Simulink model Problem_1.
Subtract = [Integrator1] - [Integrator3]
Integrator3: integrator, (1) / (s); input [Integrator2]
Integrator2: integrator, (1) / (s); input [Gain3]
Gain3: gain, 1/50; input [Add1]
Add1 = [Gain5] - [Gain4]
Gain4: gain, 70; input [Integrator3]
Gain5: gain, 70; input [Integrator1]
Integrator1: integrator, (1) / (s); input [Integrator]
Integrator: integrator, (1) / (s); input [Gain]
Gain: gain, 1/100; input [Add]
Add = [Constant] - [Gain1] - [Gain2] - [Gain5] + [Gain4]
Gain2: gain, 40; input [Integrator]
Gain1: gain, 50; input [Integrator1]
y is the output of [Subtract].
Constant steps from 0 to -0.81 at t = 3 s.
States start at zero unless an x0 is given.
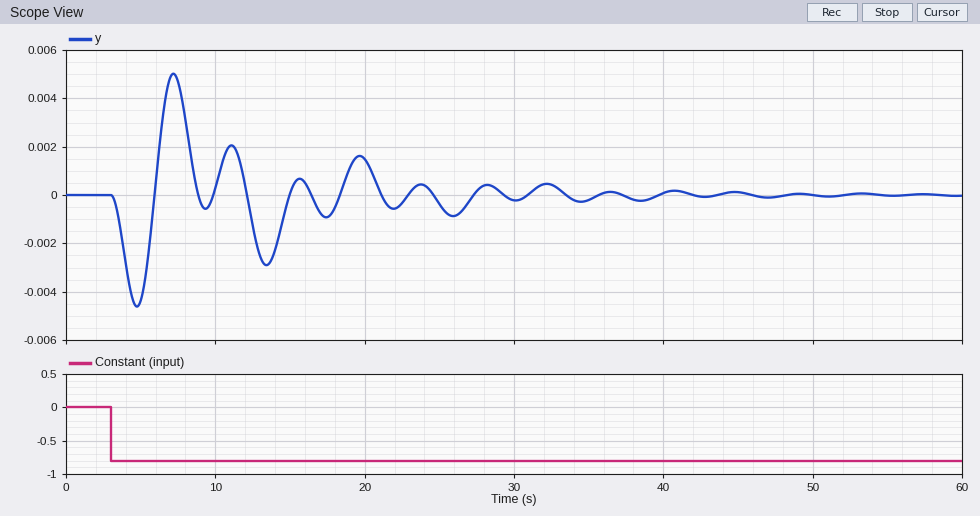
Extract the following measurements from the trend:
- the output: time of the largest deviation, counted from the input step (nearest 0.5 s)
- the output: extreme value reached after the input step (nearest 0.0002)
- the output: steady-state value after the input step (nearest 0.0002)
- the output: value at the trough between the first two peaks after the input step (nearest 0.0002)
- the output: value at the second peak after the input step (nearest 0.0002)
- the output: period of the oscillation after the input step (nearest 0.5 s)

4.0 s
0.0050
0.0000
-0.0006
0.0020
4.0 s
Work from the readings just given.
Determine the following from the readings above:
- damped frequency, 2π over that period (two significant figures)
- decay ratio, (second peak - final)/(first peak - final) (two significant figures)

1.6 rad/s
0.40
